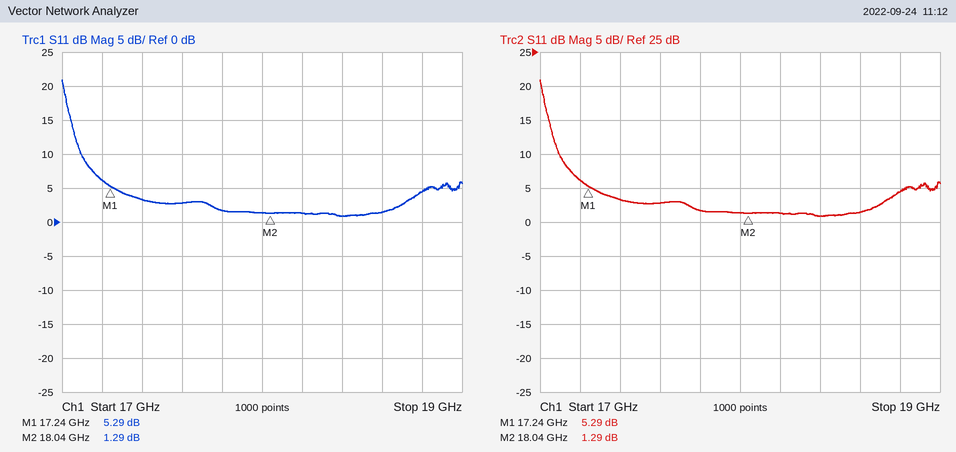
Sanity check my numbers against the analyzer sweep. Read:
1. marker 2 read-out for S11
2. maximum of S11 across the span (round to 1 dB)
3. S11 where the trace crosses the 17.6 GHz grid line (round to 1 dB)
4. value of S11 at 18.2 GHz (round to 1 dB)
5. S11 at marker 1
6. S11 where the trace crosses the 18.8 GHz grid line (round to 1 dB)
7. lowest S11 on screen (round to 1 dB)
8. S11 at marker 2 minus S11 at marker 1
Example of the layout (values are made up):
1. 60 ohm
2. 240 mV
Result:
1. 1.29 dB
2. 21 dB
3. 3 dB
4. 1 dB
5. 5.29 dB
6. 4 dB
7. 1 dB
8. -4.00 dB
